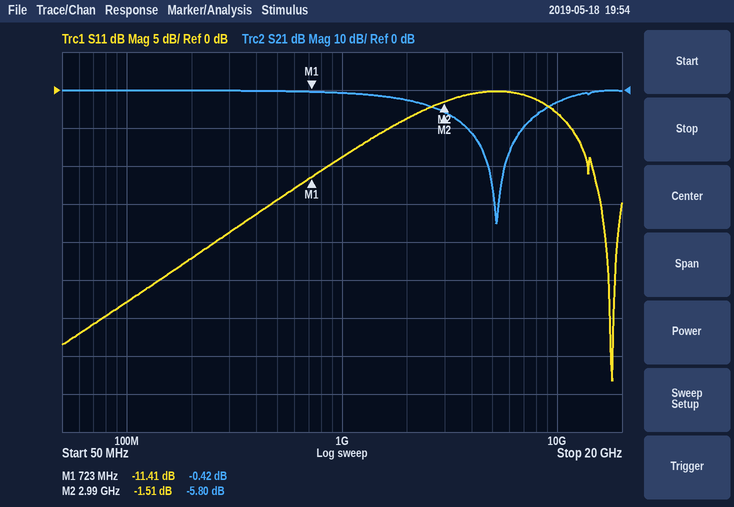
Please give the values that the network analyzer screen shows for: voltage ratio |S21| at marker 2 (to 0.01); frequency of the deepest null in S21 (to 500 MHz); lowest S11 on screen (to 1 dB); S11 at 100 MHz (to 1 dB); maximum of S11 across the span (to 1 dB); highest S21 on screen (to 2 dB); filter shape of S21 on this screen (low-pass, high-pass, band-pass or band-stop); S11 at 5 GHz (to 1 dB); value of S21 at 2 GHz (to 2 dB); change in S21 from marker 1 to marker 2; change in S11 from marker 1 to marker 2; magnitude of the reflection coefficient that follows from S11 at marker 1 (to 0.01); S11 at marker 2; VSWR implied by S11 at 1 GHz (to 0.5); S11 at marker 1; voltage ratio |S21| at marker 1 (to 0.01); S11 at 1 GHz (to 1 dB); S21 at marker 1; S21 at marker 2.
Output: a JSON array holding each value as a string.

["0.51", "5.0 GHz", "-38 dB", "-28 dB", "0 dB", "0 dB", "band-stop", "0 dB", "-2 dB", "-5.38 dB", "9.90 dB", "0.27", "-1.51 dB", "2.0", "-11.41 dB", "0.95", "-9 dB", "-0.42 dB", "-5.80 dB"]
